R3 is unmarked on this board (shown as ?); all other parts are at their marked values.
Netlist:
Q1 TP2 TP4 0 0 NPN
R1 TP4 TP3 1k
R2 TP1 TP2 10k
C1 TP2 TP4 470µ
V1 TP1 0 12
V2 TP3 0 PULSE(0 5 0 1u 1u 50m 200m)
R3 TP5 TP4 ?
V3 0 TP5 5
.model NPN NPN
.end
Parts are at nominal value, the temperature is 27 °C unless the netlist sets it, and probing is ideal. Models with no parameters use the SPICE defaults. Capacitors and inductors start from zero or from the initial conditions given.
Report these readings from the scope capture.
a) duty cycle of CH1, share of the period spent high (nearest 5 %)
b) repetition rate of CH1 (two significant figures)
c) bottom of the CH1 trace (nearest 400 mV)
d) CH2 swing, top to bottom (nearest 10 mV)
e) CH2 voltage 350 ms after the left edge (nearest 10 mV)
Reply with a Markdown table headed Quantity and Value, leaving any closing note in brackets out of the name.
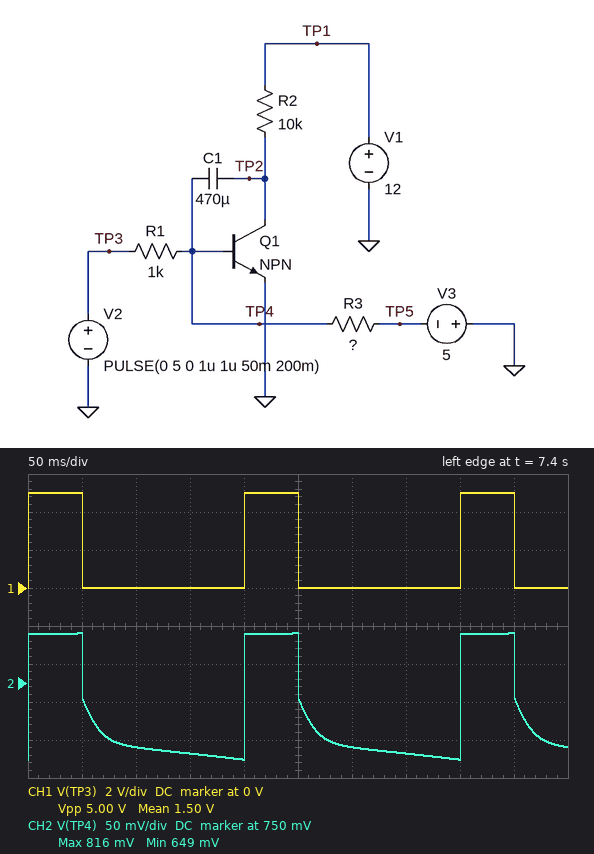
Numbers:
| Quantity | Value |
|---|---|
| duty cycle of CH1, share of the period spent high | 25 % |
| repetition rate of CH1 | 5.0 Hz |
| bottom of the CH1 trace | 0 V |
| CH2 swing, top to bottom | 170 mV |
| CH2 voltage 350 ms after the left edge | 660 mV |
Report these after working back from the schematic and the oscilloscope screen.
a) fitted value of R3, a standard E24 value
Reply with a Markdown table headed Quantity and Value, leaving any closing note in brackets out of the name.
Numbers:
| Quantity | Value |
|---|---|
| fitted value of R3, a standard E24 value | 11 kΩ |
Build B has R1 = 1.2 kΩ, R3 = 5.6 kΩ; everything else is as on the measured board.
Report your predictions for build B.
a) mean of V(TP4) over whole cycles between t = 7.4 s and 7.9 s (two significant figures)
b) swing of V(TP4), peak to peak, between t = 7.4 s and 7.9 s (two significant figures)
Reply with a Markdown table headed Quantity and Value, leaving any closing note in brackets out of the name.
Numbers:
| Quantity | Value |
|---|---|
| mean of V(TP4) over whole cycles between t = 7.4 s and 7.9 s | 230 mV |
| swing of V(TP4), peak to peak, between t = 7.4 s and 7.9 s | 780 mV |
